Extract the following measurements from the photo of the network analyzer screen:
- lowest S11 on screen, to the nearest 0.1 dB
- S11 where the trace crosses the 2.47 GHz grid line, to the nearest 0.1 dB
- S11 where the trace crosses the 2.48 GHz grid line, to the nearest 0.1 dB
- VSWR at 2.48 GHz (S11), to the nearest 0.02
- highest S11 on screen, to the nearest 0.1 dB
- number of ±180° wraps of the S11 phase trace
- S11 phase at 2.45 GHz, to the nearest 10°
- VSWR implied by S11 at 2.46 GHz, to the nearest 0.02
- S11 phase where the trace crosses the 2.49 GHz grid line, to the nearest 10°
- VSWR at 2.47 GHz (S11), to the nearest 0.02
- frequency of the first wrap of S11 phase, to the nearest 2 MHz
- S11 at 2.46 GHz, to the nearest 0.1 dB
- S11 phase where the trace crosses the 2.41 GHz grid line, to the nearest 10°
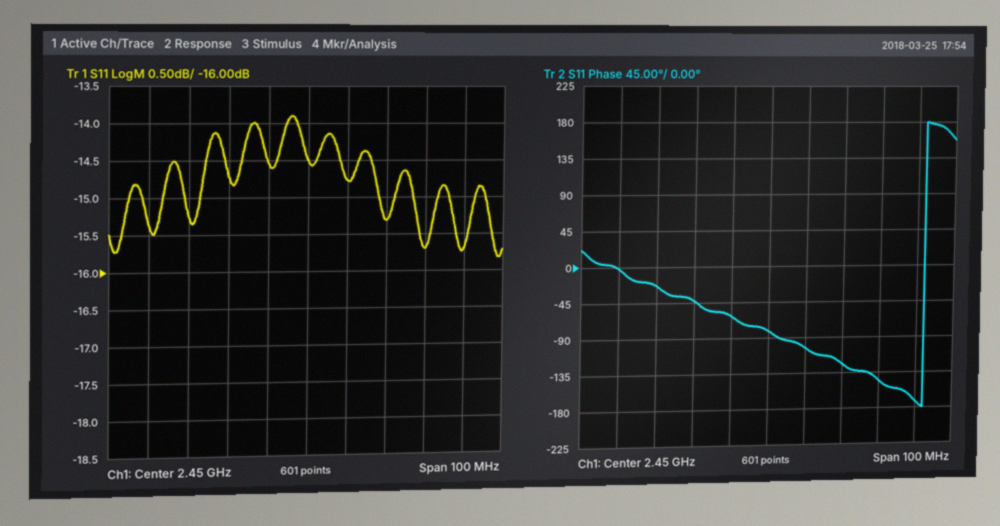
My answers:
-15.8 dB
-15.3 dB
-15.7 dB
1.40
-13.9 dB
1
-80°
1.44
-170°
1.42
2.492 GHz
-14.8 dB
0°
